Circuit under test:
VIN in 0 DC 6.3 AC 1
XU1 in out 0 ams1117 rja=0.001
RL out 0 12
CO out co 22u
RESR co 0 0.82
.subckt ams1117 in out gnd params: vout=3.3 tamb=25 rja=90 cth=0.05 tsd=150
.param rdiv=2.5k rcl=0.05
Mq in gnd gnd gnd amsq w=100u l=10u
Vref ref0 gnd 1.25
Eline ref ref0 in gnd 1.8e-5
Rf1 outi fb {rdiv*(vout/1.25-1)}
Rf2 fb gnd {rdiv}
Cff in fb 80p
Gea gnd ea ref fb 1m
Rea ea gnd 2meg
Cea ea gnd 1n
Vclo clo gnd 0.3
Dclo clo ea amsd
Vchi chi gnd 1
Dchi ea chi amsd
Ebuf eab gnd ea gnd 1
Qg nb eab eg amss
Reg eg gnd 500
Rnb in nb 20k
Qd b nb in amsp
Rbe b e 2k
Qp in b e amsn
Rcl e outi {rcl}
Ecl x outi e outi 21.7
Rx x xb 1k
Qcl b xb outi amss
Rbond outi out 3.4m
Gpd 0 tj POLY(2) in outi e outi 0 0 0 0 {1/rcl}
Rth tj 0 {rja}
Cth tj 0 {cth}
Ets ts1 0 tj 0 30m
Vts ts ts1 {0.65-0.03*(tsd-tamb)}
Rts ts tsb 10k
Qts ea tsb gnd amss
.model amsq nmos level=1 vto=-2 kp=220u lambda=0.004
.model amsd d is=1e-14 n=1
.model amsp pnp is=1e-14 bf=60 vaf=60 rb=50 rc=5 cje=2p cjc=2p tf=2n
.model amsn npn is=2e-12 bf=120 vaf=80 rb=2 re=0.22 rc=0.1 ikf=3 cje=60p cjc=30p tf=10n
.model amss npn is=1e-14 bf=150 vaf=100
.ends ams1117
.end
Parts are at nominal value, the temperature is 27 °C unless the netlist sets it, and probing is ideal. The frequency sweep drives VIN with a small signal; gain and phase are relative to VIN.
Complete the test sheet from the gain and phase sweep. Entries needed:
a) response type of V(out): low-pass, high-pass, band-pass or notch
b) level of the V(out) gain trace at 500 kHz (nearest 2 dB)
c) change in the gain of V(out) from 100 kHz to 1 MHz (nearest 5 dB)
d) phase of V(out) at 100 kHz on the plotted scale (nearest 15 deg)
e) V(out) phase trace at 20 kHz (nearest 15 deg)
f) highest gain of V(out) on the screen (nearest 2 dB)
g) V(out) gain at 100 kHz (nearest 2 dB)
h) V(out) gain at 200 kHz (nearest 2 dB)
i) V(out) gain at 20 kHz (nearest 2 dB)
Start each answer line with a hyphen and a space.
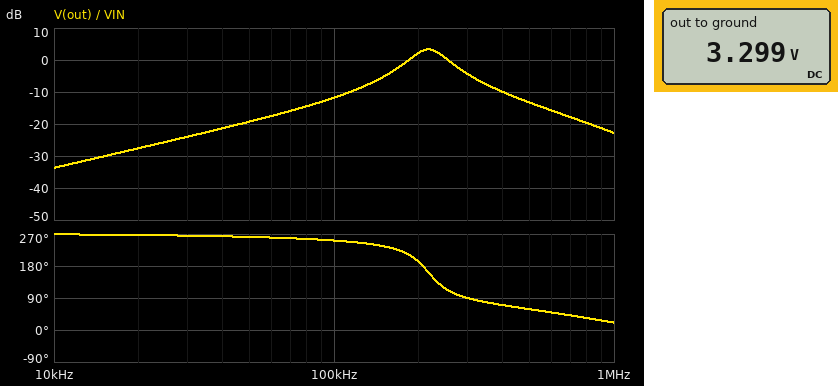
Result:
- band-pass
- -14 dB
- -10 dB
- 255 deg
- 270 deg
- 4 dB
- -12 dB
- 2 dB
- -28 dB
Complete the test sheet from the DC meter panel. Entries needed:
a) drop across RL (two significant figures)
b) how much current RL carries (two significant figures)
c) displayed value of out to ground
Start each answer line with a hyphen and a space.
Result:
- 3.3 V
- 270 mA
- 3.299 V
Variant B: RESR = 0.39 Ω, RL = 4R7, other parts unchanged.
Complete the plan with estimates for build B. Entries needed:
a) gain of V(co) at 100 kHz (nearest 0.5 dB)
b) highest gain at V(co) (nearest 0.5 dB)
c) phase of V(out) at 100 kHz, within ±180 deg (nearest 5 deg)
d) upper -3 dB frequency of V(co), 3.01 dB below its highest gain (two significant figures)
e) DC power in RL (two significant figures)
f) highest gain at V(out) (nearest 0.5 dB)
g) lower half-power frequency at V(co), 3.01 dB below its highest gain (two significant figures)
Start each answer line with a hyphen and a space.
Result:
- -27.0 dB
- -26.5 dB
- 170 deg
- 630 kHz
- 2.3 W
- -25.0 dB
- 18 kHz
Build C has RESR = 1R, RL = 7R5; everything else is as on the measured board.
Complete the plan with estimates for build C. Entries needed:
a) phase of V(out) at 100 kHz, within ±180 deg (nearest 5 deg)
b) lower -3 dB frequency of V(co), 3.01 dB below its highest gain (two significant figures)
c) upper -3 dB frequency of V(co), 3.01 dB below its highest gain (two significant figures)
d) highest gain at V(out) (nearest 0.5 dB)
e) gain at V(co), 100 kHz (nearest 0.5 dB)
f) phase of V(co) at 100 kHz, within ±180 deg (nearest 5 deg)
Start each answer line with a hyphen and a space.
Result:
- -105 deg
- 220 kHz
- 280 kHz
- 6.0 dB
- -12.5 dB
- -100 deg
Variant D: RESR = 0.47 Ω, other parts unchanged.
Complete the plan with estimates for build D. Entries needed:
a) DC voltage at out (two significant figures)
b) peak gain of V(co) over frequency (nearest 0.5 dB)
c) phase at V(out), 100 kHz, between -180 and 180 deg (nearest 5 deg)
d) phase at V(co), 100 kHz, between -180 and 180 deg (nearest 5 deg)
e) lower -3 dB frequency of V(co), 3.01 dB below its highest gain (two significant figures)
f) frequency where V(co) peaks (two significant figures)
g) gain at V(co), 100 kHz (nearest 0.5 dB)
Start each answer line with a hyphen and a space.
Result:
- 3.3 V
- -3.5 dB
- -125 deg
- -115 deg
- 130 kHz
- 170 kHz
- -10.5 dB
